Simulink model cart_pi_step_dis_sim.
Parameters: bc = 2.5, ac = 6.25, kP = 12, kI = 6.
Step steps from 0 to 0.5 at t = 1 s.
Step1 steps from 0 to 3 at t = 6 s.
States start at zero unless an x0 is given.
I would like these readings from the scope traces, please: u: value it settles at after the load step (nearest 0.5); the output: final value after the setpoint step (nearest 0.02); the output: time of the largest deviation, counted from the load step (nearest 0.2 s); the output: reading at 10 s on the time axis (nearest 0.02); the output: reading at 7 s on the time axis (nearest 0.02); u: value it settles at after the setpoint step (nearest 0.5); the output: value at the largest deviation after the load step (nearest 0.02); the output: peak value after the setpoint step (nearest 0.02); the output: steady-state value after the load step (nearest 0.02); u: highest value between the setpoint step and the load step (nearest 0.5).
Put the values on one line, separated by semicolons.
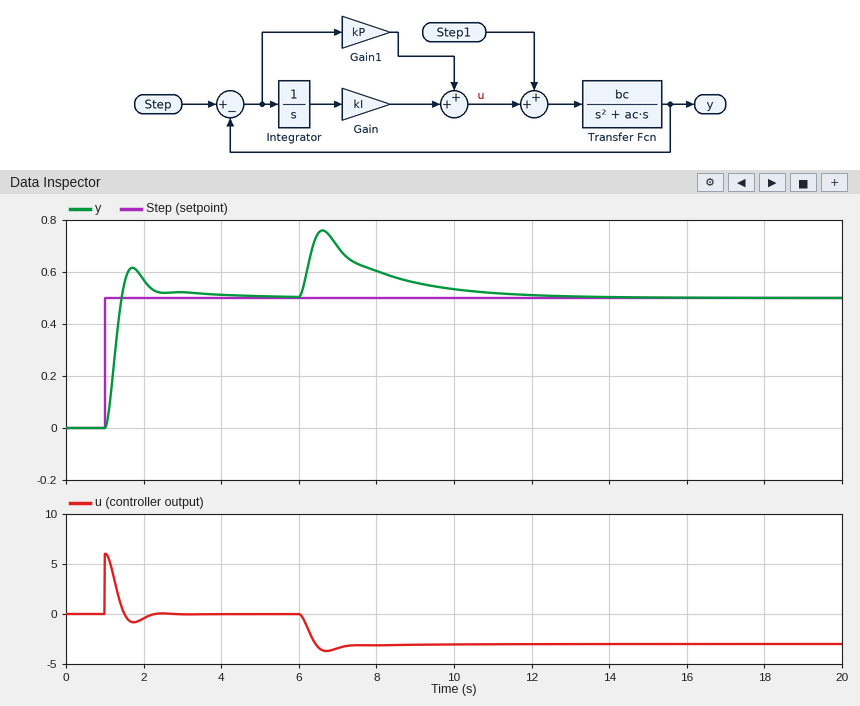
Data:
-3.0; 0.50; 0.6 s; 0.54; 0.70; 0.0; 0.76; 0.62; 0.50; 6.0
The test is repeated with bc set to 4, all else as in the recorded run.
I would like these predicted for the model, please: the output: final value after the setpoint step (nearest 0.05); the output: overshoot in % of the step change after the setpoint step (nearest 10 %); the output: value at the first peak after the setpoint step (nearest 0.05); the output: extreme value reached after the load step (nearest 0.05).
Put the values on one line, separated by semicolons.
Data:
0.50; 30 %; 0.65; 0.80
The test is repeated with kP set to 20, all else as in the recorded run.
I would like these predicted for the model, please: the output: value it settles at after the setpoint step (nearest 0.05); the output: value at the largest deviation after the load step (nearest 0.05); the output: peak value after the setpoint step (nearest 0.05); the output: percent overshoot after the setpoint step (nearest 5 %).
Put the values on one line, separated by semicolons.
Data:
0.50; 0.70; 0.65; 25 %
